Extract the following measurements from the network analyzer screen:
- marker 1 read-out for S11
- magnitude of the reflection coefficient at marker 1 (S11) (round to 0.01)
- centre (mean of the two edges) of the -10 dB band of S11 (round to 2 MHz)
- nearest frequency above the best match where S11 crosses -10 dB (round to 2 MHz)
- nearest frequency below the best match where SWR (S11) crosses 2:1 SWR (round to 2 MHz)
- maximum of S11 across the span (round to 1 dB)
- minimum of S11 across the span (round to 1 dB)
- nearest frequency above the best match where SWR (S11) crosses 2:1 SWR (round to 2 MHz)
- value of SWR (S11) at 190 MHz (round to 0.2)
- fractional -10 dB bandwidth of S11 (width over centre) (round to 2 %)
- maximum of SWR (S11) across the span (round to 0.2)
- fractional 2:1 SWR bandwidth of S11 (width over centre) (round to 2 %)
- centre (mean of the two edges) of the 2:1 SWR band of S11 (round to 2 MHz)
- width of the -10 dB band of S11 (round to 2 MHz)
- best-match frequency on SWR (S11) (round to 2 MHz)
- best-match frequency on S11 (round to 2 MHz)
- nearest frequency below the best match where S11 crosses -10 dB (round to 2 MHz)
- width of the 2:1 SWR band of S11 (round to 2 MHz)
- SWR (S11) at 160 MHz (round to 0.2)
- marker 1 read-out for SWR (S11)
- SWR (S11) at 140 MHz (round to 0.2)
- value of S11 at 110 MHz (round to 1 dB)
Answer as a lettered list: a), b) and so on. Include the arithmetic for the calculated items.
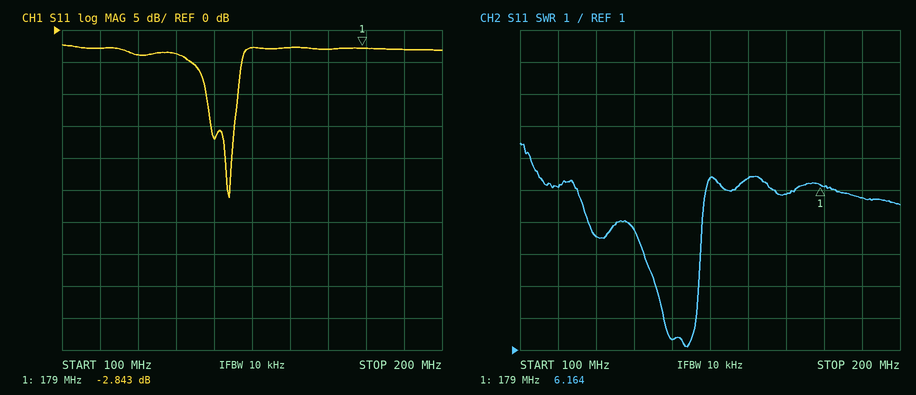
a) -2.843 dB
b) 10^(-2.843/20) ≈ 0.72
c) 142 MHz
d) 146 MHz
e) 138 MHz
f) -2 dB
g) -26 dB
h) 146 MHz
i) 5.8
j) 8 MHz / 142 MHz ≈ 6 %
k) 7.4
l) 8 MHz / 142 MHz ≈ 6 %
m) 142 MHz
n) 146 MHz − 138 MHz = 8 MHz
o) 144 MHz
p) 144 MHz
q) 138 MHz
r) 146 MHz − 138 MHz = 8 MHz
s) 6.4
t) 6.164
u) 1.4
v) -3 dB
